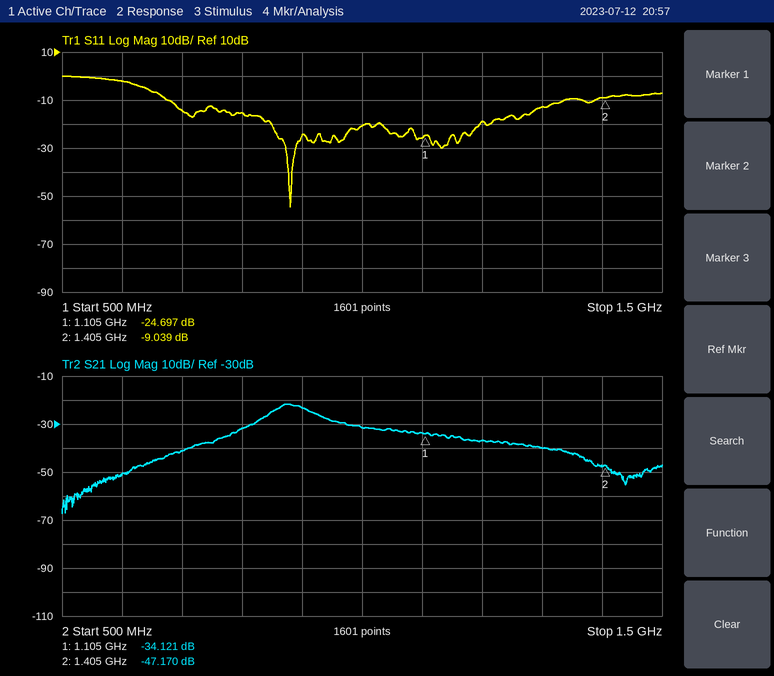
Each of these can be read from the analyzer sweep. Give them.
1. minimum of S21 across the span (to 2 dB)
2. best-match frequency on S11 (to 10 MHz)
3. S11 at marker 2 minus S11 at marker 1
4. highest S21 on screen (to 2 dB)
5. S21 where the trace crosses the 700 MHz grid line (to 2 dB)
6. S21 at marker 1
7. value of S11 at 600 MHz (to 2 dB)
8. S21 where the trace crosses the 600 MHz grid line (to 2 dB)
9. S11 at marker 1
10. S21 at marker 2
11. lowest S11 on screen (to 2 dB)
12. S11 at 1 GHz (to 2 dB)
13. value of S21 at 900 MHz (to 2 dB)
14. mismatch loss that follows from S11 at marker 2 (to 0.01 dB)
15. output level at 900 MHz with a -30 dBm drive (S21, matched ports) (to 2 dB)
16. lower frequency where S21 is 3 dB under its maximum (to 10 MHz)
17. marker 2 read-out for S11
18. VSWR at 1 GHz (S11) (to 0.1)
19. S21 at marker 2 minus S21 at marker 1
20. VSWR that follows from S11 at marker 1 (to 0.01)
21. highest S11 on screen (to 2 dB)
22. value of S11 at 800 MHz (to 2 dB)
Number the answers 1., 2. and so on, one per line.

1. -68 dB
2. 880 MHz
3. 15.658 dB
4. -22 dB
5. -42 dB
6. -34.121 dB
7. -2 dB
8. -50 dB
9. -24.697 dB
10. -47.170 dB
11. -54 dB
12. -20 dB
13. -24 dB
14. 0.58 dB
15. -54 dBm
16. 850 MHz
17. -9.039 dB
18. 1.2
19. -13.049 dB
20. 1.12
21. 0 dB
22. -16 dB
